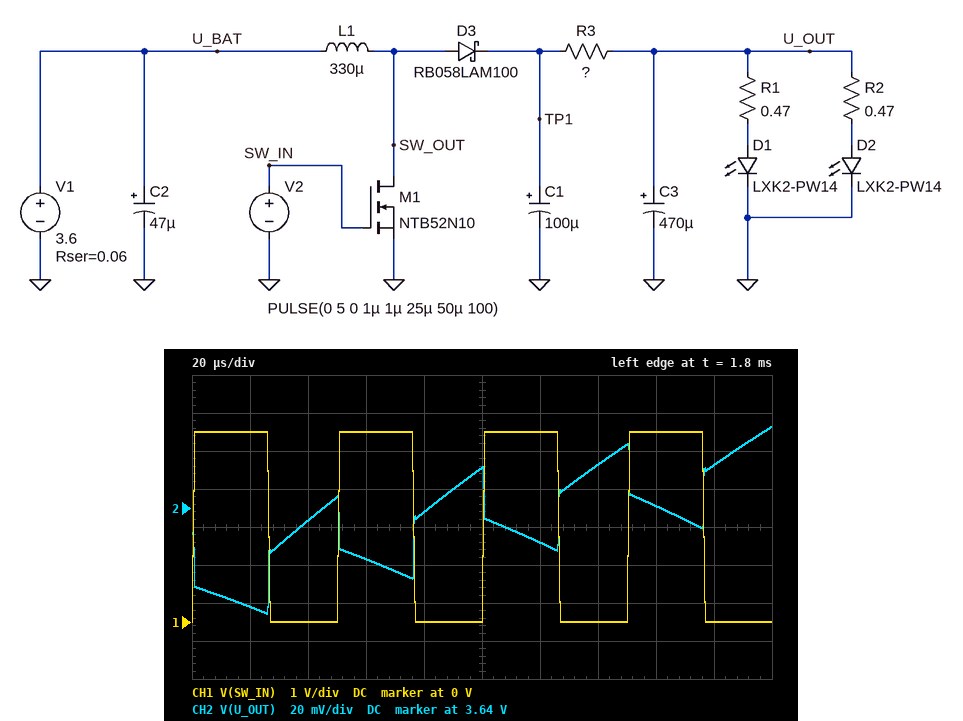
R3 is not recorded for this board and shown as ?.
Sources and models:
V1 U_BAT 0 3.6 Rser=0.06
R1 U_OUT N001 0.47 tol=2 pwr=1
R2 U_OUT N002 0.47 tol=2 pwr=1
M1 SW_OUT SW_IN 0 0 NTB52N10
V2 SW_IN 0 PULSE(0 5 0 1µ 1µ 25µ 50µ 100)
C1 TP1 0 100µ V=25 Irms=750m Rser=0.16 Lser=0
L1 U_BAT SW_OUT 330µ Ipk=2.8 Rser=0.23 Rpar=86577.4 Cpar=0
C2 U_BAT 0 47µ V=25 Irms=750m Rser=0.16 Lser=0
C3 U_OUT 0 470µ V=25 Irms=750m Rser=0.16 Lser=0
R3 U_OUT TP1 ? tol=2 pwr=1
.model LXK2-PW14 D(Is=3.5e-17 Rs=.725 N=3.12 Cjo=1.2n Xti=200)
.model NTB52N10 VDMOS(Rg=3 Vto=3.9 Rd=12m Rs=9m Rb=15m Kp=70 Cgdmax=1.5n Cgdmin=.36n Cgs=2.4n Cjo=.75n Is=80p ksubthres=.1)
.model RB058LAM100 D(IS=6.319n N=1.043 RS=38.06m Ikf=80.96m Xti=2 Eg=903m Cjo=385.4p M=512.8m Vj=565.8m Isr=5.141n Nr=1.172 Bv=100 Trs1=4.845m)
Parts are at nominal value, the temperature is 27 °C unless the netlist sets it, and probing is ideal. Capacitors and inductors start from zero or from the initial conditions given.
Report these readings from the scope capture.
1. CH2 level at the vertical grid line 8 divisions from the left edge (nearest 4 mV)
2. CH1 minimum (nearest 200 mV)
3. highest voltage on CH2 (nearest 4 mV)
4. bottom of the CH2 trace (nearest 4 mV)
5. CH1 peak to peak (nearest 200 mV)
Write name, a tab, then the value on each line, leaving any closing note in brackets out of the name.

CH2 level at the vertical grid line 8 divisions from the left edge	3.640 V
CH1 minimum	0 V
highest voltage on CH2	3.684 V
bottom of the CH2 trace	3.584 V
CH1 peak to peak	5.0 V
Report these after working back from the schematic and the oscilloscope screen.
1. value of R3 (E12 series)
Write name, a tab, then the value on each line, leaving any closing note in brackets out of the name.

value of R3	1.5 Ω
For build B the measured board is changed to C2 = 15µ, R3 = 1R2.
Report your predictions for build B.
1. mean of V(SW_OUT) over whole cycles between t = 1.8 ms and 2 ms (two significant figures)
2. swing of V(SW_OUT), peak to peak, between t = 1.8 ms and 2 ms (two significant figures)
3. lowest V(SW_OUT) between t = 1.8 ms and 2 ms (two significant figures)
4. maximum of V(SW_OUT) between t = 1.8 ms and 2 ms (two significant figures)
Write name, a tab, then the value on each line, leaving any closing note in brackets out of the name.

mean of V(SW_OUT) over whole cycles between t = 1.8 ms and 2 ms	3.1 V
swing of V(SW_OUT), peak to peak, between t = 1.8 ms and 2 ms	6.3 V
lowest V(SW_OUT) between t = 1.8 ms and 2 ms	88 mV
maximum of V(SW_OUT) between t = 1.8 ms and 2 ms	6.4 V
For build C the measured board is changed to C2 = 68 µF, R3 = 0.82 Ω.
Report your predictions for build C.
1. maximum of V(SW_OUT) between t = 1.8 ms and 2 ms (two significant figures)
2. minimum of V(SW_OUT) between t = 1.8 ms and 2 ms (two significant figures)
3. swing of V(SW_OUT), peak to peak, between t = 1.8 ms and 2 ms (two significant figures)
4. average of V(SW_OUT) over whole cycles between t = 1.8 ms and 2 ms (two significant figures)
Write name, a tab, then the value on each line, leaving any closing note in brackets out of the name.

maximum of V(SW_OUT) between t = 1.8 ms and 2 ms	6.2 V
minimum of V(SW_OUT) between t = 1.8 ms and 2 ms	100 mV
swing of V(SW_OUT), peak to peak, between t = 1.8 ms and 2 ms	6.1 V
average of V(SW_OUT) over whole cycles between t = 1.8 ms and 2 ms	3.0 V
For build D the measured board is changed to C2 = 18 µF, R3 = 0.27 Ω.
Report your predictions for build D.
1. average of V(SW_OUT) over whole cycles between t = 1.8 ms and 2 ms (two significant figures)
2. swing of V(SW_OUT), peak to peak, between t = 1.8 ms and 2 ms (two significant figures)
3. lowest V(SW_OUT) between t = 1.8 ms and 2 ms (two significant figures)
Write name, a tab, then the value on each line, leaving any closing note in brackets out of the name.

average of V(SW_OUT) over whole cycles between t = 1.8 ms and 2 ms	2.8 V
swing of V(SW_OUT), peak to peak, between t = 1.8 ms and 2 ms	5.5 V
lowest V(SW_OUT) between t = 1.8 ms and 2 ms	120 mV
